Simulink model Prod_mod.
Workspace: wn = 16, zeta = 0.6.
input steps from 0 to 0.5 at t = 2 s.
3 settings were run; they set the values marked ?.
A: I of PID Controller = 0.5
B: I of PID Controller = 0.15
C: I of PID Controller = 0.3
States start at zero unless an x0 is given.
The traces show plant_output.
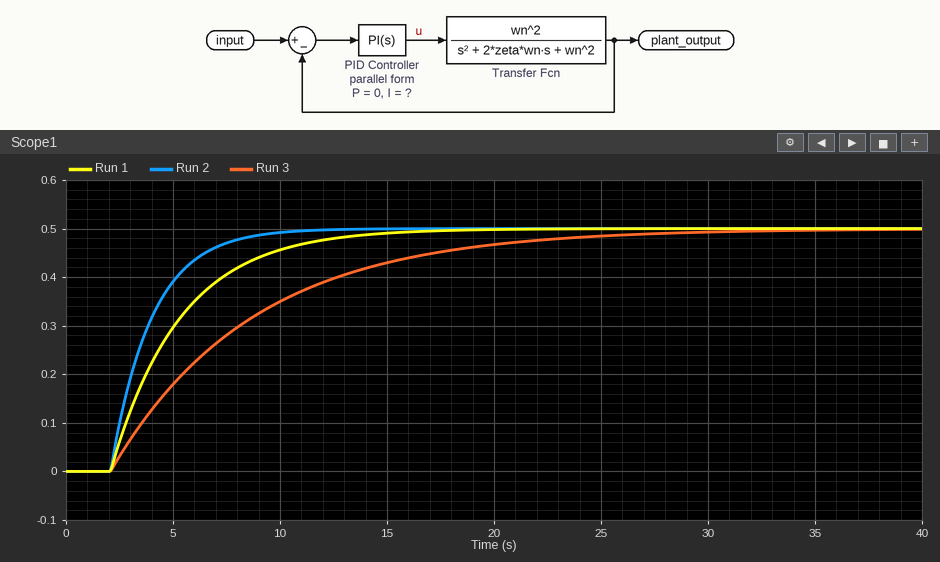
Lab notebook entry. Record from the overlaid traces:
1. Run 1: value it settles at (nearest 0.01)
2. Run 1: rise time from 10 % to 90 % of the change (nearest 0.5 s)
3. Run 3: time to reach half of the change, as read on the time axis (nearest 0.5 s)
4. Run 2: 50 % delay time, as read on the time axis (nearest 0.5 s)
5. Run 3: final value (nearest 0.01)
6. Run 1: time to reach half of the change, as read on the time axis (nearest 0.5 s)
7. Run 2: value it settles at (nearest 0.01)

0.50
7.0 s
6.5 s
3.5 s
0.50
4.5 s
0.50
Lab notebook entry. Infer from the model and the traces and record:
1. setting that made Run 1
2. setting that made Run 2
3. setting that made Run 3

C
A
B
